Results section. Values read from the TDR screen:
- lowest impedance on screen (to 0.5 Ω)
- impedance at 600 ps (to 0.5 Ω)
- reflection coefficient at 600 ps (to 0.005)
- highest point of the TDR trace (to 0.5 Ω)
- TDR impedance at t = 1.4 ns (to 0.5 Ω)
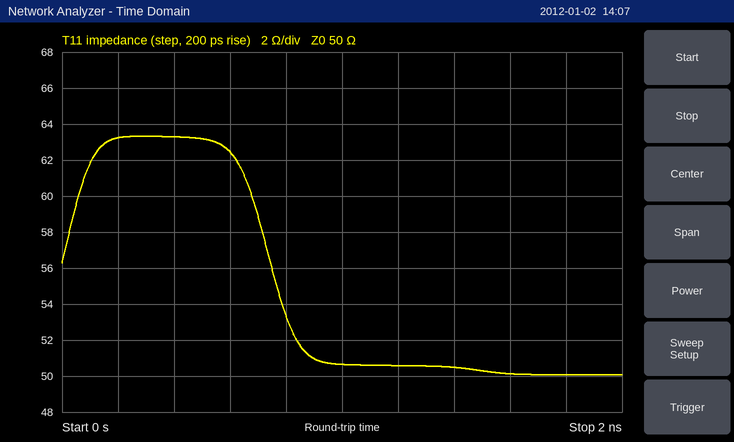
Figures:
50.0 Ω
62.5 Ω
+0.110
63.5 Ω
50.5 Ω
